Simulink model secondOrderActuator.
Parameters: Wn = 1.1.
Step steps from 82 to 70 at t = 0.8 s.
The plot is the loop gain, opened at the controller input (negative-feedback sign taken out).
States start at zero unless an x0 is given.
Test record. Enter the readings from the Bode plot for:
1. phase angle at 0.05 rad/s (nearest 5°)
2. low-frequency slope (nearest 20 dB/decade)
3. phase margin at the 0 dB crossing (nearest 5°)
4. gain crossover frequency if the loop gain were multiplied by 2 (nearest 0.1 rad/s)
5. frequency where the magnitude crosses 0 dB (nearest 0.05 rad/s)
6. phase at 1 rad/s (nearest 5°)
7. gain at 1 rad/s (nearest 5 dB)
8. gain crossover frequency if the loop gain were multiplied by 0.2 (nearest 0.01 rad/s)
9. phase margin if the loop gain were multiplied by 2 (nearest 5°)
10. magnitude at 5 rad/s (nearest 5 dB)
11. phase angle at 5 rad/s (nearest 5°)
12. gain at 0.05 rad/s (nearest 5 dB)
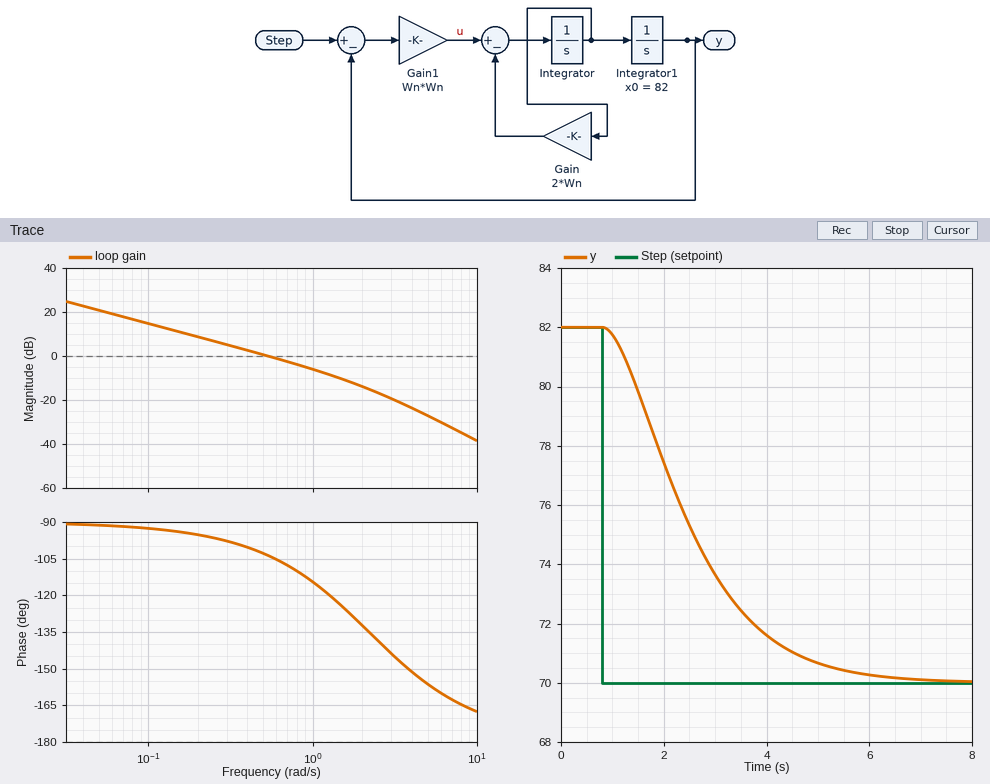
-90°
-20 dB/decade
75°
1.0 rad/s
0.55 rad/s
-115°
-5 dB
0.11 rad/s
65°
-25 dB
-155°
20 dB
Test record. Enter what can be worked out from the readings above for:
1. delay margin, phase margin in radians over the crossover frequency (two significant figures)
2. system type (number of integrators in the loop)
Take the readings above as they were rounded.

2.4 s
1
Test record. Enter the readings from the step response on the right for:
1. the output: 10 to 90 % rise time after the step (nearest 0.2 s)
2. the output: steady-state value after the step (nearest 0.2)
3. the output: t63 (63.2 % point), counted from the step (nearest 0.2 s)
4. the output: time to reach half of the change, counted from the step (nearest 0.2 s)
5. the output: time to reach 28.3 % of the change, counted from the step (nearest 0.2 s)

3.0 s
70.0
2.0 s
1.6 s
1.0 s
